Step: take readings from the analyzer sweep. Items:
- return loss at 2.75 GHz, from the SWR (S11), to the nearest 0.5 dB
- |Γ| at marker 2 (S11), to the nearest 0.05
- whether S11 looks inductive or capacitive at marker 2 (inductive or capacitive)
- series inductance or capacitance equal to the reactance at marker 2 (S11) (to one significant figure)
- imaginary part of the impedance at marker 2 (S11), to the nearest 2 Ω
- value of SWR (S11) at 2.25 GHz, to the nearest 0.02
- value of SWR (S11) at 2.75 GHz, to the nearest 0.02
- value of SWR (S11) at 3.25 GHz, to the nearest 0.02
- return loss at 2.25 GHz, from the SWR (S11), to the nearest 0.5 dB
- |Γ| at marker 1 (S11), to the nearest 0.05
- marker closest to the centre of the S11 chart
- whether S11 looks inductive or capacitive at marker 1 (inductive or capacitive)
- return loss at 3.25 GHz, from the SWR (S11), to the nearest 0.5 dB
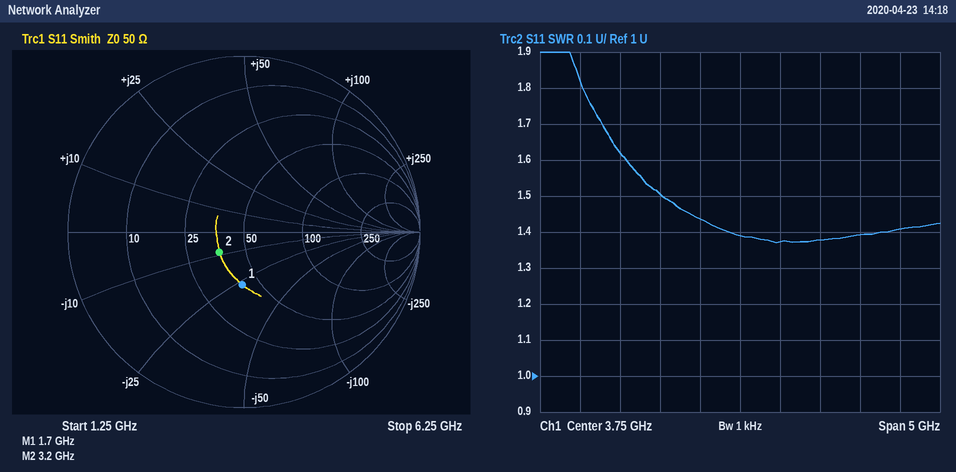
14.0 dB
0.20
capacitive
6 pF
-8 Ω
1.62
1.50
1.44
12.5 dB
0.30
marker 2
capacitive
15.0 dB
